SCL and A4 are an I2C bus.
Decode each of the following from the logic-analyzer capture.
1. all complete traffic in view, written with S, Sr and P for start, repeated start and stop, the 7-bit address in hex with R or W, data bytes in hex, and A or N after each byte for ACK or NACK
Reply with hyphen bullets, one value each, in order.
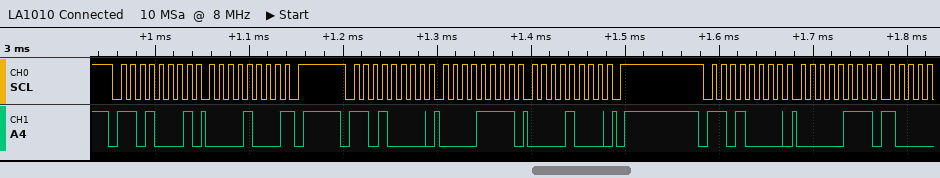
- S 68R A 08 N P S 68W A 0F A 08 A P S 68W A 07 A
